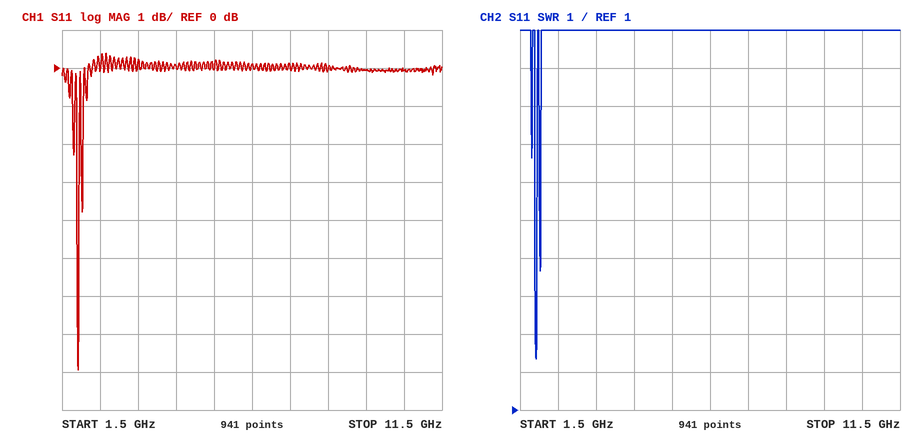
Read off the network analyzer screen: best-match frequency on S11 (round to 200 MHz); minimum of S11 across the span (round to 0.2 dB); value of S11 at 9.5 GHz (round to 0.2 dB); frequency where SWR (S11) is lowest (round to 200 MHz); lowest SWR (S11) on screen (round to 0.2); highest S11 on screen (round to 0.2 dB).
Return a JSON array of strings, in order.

["2.0 GHz", "-8.0 dB", "0.0 dB", "2.0 GHz", "2.4", "0.4 dB"]
